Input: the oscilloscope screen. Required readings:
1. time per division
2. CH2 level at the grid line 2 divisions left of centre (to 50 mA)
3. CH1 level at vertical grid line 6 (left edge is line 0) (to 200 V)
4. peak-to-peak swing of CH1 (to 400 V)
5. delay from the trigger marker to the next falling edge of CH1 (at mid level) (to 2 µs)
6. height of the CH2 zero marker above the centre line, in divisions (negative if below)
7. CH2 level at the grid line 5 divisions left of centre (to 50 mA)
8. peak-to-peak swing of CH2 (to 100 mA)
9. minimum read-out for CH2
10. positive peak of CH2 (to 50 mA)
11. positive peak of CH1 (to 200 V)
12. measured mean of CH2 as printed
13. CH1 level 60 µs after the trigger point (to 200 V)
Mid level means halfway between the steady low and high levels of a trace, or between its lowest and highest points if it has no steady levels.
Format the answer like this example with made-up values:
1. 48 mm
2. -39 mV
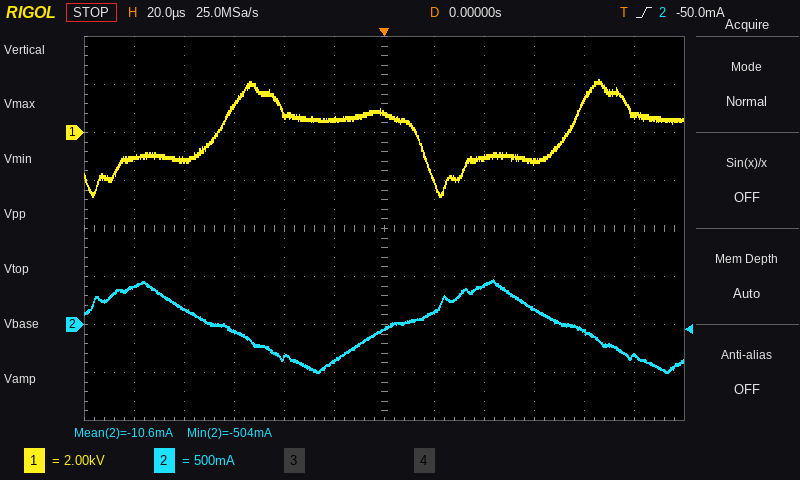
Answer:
1. 20 µs
2. -350 mA
3. 800 V
4. 4.8 kV
5. 14 µs
6. -2.0 div
7. 400 mA
8. 1.00 A
9. -504 mA
10. 450 mA
11. 2.2 kV
12. -10.6 mA
13. -1.2 kV
